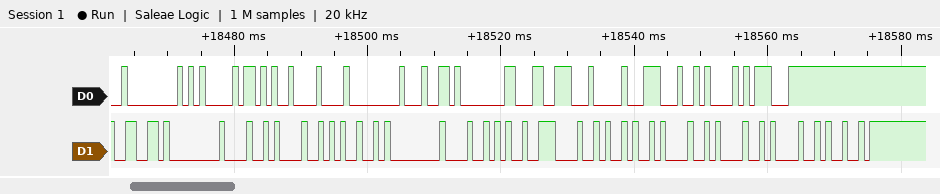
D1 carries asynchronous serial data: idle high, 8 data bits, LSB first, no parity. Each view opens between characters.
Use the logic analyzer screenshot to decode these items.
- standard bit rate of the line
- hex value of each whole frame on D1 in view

1200 baud
66, 00, 48, 48, 49, 00, 48, C9, 48, 4A, 48, 48, 48, D2
